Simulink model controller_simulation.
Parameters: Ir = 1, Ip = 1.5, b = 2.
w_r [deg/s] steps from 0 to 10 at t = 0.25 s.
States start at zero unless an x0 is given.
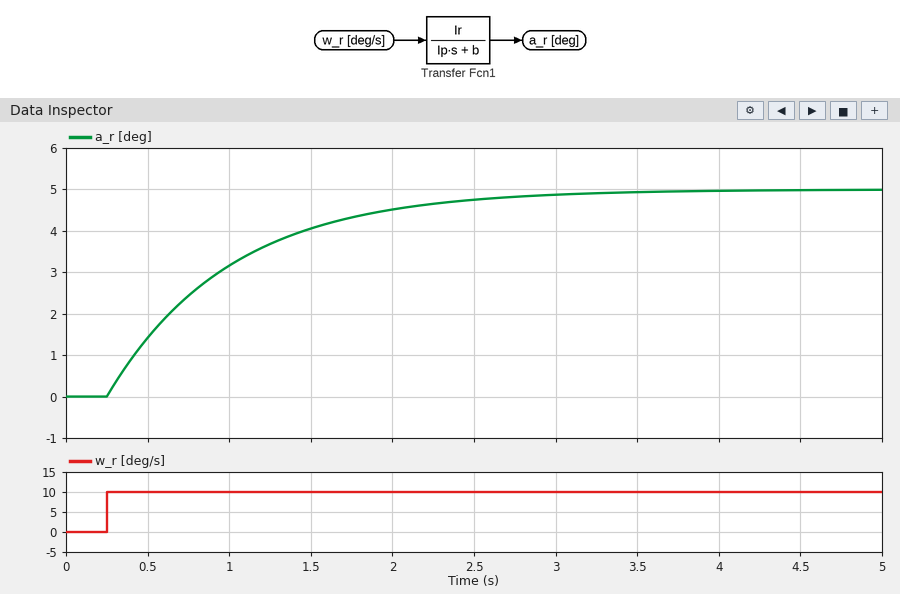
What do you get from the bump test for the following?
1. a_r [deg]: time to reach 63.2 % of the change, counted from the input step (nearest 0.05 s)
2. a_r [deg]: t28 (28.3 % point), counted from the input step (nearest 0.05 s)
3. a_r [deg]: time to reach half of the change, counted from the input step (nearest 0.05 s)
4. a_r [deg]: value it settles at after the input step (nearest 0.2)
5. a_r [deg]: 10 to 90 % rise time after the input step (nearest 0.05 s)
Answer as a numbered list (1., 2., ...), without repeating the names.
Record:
1. 0.75 s
2. 0.25 s
3. 0.50 s
4. 5.0
5. 1.65 s
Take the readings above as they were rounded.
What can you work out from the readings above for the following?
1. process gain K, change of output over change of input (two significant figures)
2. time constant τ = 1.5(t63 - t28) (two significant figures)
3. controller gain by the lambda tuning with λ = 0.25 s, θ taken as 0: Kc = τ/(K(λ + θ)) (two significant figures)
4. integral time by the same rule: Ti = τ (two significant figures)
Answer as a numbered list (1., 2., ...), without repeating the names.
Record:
1. 0.50
2. 0.75 s
3. 6.0
4. 0.75 s
